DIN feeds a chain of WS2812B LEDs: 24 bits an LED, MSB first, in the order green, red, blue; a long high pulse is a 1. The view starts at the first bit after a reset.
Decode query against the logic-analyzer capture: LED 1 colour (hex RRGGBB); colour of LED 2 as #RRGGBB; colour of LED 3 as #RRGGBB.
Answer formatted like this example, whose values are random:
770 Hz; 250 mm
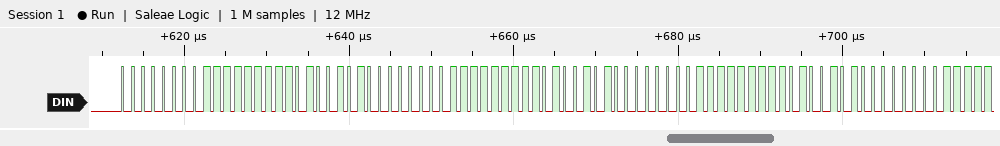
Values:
#FF00A5; #FF00A5; #FF00A5
